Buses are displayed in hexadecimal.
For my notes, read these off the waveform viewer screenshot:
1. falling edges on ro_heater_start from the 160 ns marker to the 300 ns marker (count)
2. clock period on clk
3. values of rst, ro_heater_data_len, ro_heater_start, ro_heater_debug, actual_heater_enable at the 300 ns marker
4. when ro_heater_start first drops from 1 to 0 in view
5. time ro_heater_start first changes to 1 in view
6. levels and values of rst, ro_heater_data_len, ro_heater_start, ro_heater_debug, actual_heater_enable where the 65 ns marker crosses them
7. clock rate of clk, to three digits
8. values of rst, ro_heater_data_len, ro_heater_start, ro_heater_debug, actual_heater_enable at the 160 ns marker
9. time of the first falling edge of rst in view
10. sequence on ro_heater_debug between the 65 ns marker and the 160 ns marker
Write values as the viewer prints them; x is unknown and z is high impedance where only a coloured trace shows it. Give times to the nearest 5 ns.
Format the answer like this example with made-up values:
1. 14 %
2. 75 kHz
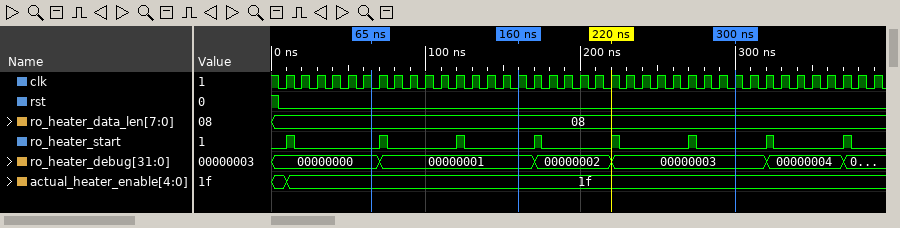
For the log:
1. 3
2. 10 ns
3. rst=0, ro_heater_data_len=08, ro_heater_start=0, ro_heater_debug=00000003, actual_heater_enable=1f
4. 15 ns
5. 10 ns
6. rst=0, ro_heater_data_len=08, ro_heater_start=0, ro_heater_debug=00000000, actual_heater_enable=1f
7. 100 MHz
8. rst=0, ro_heater_data_len=08, ro_heater_start=0, ro_heater_debug=00000001, actual_heater_enable=1f
9. 5 ns
10. 00000000, 00000001
